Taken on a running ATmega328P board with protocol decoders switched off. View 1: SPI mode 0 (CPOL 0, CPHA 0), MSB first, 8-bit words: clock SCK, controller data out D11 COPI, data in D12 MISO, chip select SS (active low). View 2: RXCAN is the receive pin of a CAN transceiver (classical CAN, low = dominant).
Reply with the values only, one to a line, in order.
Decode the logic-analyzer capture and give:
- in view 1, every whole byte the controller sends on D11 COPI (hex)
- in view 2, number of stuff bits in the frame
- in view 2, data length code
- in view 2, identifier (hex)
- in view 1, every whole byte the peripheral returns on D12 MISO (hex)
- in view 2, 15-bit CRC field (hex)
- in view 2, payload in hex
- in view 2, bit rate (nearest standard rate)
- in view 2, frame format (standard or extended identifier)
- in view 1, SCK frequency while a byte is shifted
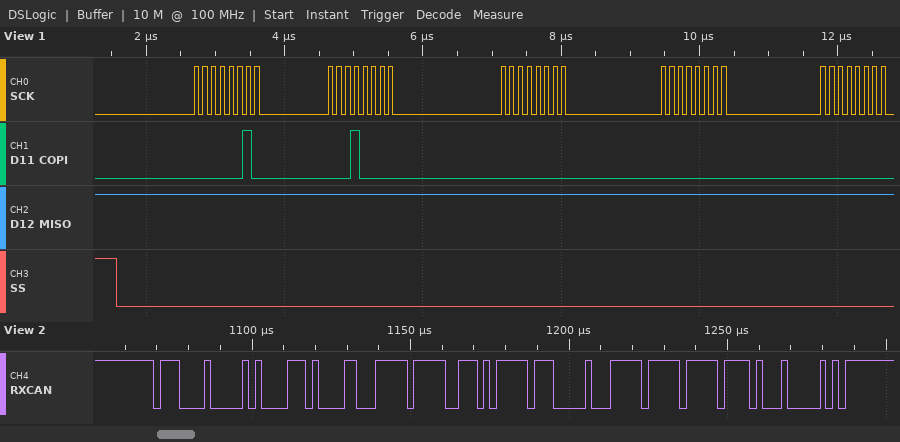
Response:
02 10 00 00 00
9
8
0x708
FF FF FF FF FF
0x7440
74 31 FF BA FF 00 FF FF
500 kbit/s
standard
8 MHz
